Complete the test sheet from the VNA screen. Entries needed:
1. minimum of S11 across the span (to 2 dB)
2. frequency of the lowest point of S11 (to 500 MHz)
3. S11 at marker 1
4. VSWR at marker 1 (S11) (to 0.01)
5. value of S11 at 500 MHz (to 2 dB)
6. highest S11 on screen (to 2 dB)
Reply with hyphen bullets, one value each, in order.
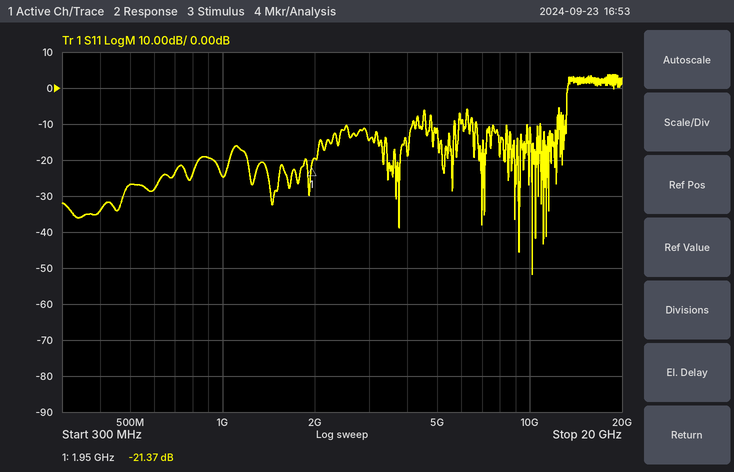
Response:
- -52 dB
- 10.0 GHz
- -21.37 dB
- 1.19
- -26 dB
- 4 dB
